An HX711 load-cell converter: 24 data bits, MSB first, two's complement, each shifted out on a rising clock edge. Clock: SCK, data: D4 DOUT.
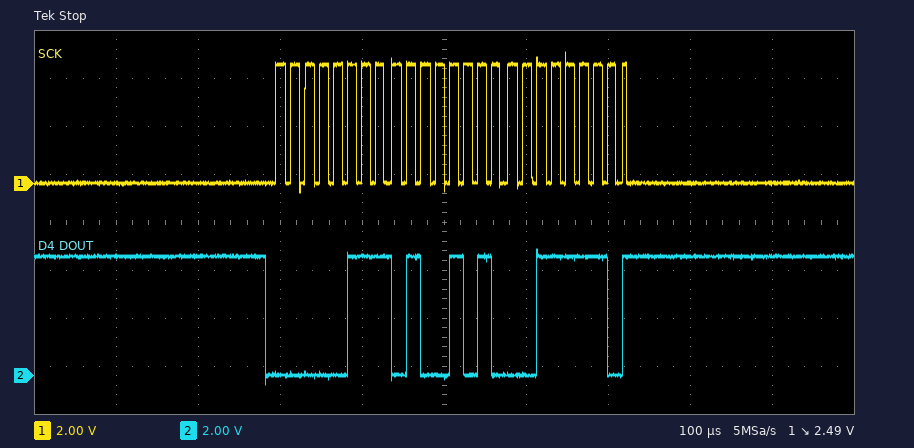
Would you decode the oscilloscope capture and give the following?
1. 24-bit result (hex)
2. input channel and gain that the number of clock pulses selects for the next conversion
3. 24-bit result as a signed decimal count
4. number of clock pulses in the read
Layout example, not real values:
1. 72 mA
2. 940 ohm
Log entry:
1. 0x074A3E
2. channel A, gain 128
3. 477758
4. 25
